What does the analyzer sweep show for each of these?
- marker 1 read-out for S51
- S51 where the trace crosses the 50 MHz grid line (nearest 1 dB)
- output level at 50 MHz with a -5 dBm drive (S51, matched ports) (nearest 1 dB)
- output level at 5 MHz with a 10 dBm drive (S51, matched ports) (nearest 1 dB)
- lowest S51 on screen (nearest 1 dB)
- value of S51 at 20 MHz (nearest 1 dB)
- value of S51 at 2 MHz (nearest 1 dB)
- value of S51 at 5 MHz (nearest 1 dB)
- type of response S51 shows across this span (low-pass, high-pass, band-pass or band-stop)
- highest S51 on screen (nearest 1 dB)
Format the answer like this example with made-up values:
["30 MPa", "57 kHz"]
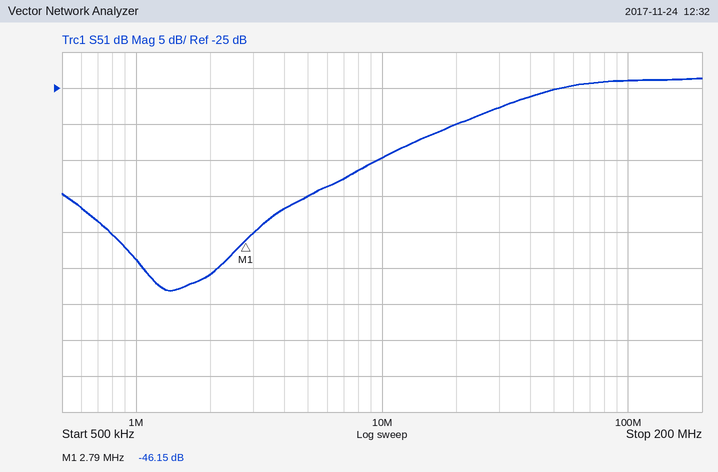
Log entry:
["-46.15 dB", "-25 dB", "-30 dBm", "-30 dBm", "-53 dB", "-30 dB", "-51 dB", "-40 dB", "high-pass", "-24 dB"]
